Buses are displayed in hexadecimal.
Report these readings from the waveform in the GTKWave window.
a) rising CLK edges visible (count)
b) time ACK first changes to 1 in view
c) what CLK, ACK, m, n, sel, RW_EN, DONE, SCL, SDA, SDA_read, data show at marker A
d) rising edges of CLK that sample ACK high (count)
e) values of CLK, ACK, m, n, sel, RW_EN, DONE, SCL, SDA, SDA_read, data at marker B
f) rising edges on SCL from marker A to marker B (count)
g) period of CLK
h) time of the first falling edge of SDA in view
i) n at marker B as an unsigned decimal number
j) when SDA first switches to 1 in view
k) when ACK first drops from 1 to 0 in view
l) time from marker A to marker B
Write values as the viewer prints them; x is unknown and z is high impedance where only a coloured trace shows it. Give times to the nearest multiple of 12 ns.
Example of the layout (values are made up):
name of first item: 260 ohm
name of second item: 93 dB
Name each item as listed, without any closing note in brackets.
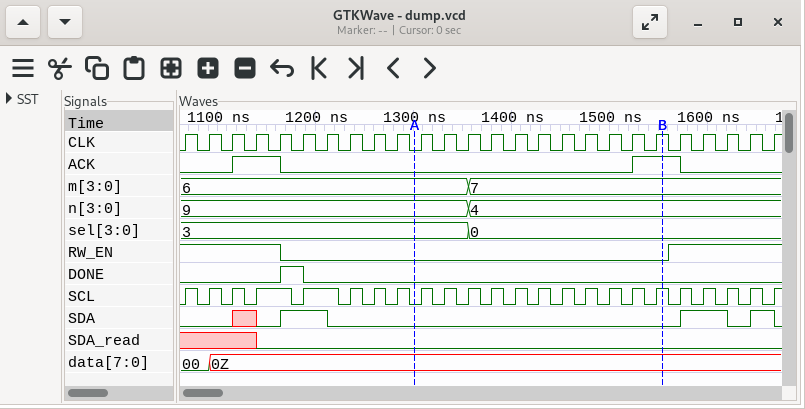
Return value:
rising CLK edges visible: 26
time ACK first changes to 1 in view: 1116 ns
what CLK, ACK, m, n, sel, RW_EN, DONE, SCL, SDA, SDA_read, data show at marker A: CLK=0, ACK=0, m=6, n=9, sel=3, RW_EN=0, DONE=0, SCL=0, SDA=0, SDA_read=0, data=0Z
rising edges of CLK that sample ACK high: 4
values of CLK, ACK, m, n, sel, RW_EN, DONE, SCL, SDA, SDA_read, data at marker B: CLK=1, ACK=1, m=7, n=4, sel=0, RW_EN=0, DONE=0, SCL=1, SDA=0, SDA_read=0, data=0Z
rising edges on SCL from marker A to marker B: 11
period of CLK: 24 ns
time of the first falling edge of SDA in view: 1212 ns
n at marker B as an unsigned decimal number: 4
when SDA first switches to 1 in view: 1164 ns
when ACK first drops from 1 to 0 in view: 1164 ns
time from marker A to marker B: 252 ns
